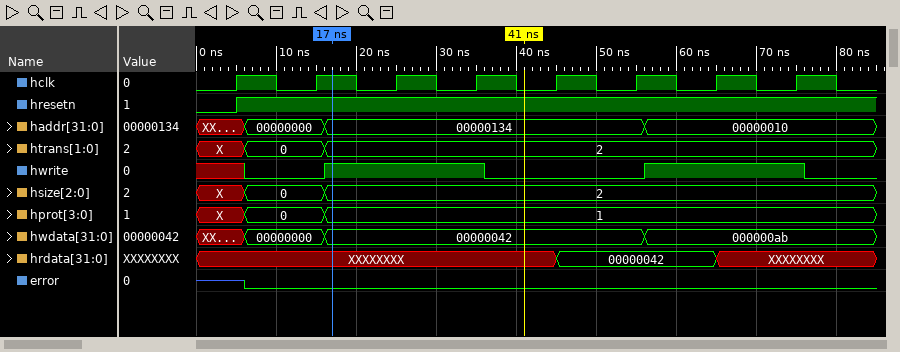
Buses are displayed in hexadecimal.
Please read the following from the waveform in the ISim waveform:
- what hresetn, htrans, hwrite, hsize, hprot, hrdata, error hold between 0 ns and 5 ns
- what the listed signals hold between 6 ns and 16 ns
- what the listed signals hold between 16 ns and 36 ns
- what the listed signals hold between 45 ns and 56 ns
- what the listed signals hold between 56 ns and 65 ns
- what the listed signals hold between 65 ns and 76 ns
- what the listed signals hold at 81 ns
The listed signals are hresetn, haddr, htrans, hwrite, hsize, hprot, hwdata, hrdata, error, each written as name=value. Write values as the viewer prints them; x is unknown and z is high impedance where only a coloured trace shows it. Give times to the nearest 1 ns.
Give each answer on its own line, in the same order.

hresetn=0, htrans=X, hwrite=x, hsize=X, hprot=X, hrdata=XXXXXXXX, error=z
hresetn=1, haddr=00000000, htrans=0, hwrite=0, hsize=0, hprot=0, hwdata=00000000, hrdata=XXXXXXXX, error=0
hresetn=1, haddr=00000134, htrans=2, hwrite=1, hsize=2, hprot=1, hwdata=00000042, hrdata=XXXXXXXX, error=0
hresetn=1, haddr=00000134, htrans=2, hwrite=0, hsize=2, hprot=1, hwdata=00000042, hrdata=00000042, error=0
hresetn=1, haddr=00000010, htrans=2, hwrite=1, hsize=2, hprot=1, hwdata=000000ab, hrdata=00000042, error=0
hresetn=1, haddr=00000010, htrans=2, hwrite=1, hsize=2, hprot=1, hwdata=000000ab, hrdata=XXXXXXXX, error=0
hresetn=1, haddr=00000010, htrans=2, hwrite=0, hsize=2, hprot=1, hwdata=000000ab, hrdata=XXXXXXXX, error=0
